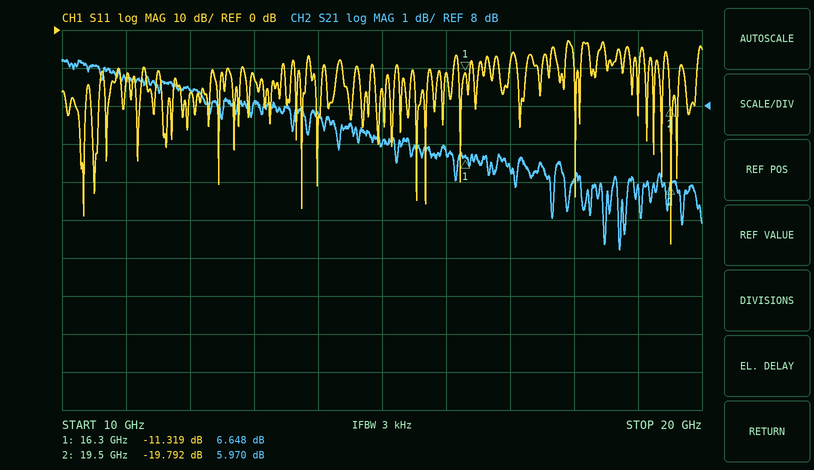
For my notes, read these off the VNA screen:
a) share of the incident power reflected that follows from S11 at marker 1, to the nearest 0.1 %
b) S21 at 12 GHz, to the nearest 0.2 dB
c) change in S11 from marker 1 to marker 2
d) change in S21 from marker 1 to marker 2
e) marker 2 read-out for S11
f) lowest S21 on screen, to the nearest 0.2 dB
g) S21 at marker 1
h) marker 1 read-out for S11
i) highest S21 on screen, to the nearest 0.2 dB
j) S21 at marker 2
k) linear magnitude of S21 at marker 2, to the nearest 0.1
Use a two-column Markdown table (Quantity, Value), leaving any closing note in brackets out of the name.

| Quantity | Value |
|---|---|
| share of the incident power reflected that follows from S11 at marker 1, to the nearest 0.1 % | 7.4 % |
| S21 at 12 GHz, to the nearest 0.2 dB | 8.4 dB |
| change in S11 from marker 1 to marker 2 | -8.473 dB |
| change in S21 from marker 1 to marker 2 | -0.678 dB |
| marker 2 read-out for S11 | -19.792 dB |
| lowest S21 on screen, to the nearest 0.2 dB | 4.2 dB |
| S21 at marker 1 | 6.648 dB |
| marker 1 read-out for S11 | -11.319 dB |
| highest S21 on screen, to the nearest 0.2 dB | 9.2 dB |
| S21 at marker 2 | 5.970 dB |
| linear magnitude of S21 at marker 2, to the nearest 0.1 | 2.0 |
